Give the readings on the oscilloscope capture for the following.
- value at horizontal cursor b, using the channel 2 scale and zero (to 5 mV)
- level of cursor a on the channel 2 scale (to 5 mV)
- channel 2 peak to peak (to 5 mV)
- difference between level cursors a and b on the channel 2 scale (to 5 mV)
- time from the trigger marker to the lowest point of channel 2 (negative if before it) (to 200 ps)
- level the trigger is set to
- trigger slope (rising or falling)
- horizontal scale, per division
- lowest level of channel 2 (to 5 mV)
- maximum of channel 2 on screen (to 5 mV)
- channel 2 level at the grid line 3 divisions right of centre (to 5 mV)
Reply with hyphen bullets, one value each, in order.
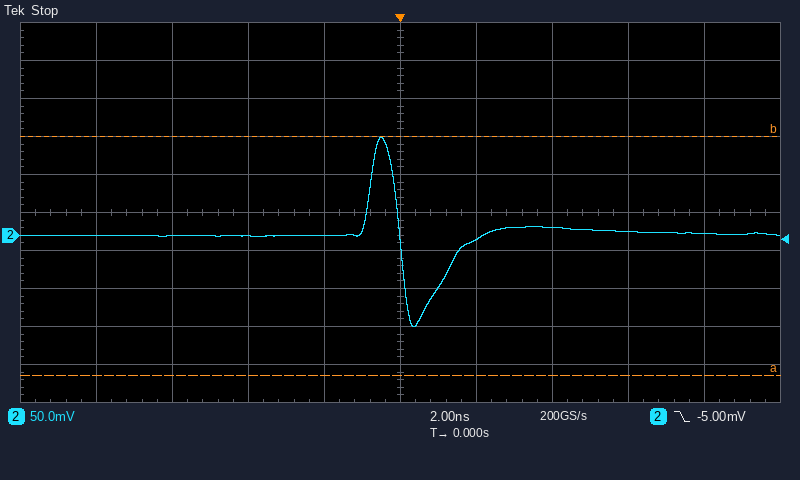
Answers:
- 130 mV
- -185 mV
- 250 mV
- 315 mV
- +400 ps
- -5.00 mV
- falling
- 2 ns
- -120 mV
- 130 mV
- 5 mV
